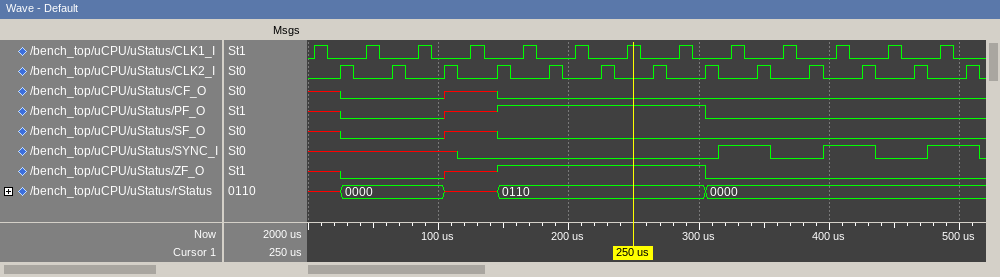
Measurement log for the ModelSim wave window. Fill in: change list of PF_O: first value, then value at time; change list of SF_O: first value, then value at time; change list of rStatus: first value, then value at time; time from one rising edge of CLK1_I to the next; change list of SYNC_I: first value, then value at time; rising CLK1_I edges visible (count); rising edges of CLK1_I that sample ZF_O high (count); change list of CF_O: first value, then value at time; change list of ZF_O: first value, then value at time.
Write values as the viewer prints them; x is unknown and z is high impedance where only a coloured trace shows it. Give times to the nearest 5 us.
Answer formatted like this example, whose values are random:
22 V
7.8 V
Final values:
x, 0 at 25 us, x at 105 us, 1 at 145 us, 0 at 305 us
x, 0 at 25 us, x at 105 us, 0 at 145 us
x, 0000 at 25 us, x at 105 us, 0110 at 145 us, 0000 at 305 us
40 us
x, 0 at 115 us, 1 at 315 us, 0 at 355 us, 1 at 395 us, 0 at 435 us, 1 at 475 us, 0 at 515 us
13
4
x, 0 at 25 us, x at 105 us, 0 at 145 us
x, 0 at 25 us, x at 105 us, 1 at 145 us, 0 at 305 us
